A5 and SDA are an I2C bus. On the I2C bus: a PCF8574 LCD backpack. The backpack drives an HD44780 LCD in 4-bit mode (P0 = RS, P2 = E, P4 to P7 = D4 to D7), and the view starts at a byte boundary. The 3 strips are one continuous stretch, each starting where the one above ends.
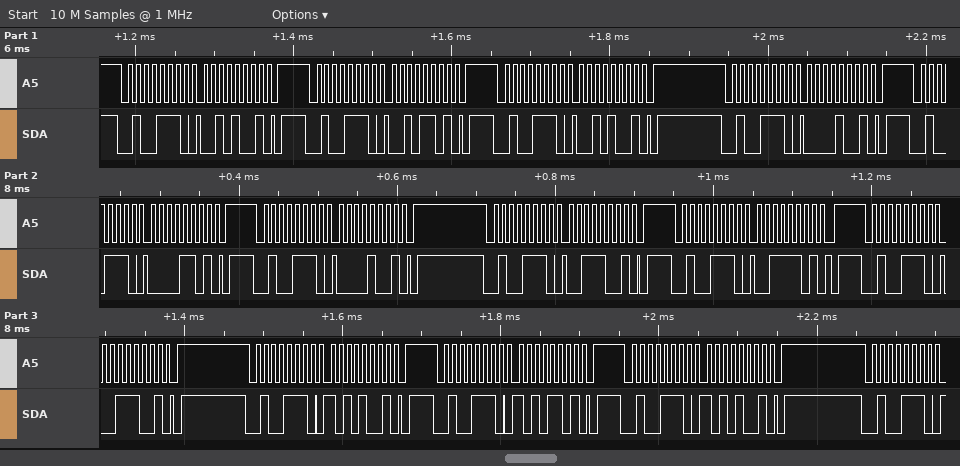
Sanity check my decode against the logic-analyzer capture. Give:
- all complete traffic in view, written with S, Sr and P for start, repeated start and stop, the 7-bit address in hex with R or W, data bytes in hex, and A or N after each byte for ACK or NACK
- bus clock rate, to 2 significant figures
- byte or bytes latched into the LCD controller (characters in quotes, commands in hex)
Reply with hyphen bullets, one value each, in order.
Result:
- S 27W A 29 A P S 27W A 2D A P S 27W A 29 A P S 27W A 09 A P S 27W A 0D A P S 27W A 09 A P S 27W A 39 A P S 27W A 3D A P S 27W A 39 A P S 27W A A9 A P S 27W A AD A P S 27W A A9 A P S 27W A
- 100 kHz
- ' ' ':'
